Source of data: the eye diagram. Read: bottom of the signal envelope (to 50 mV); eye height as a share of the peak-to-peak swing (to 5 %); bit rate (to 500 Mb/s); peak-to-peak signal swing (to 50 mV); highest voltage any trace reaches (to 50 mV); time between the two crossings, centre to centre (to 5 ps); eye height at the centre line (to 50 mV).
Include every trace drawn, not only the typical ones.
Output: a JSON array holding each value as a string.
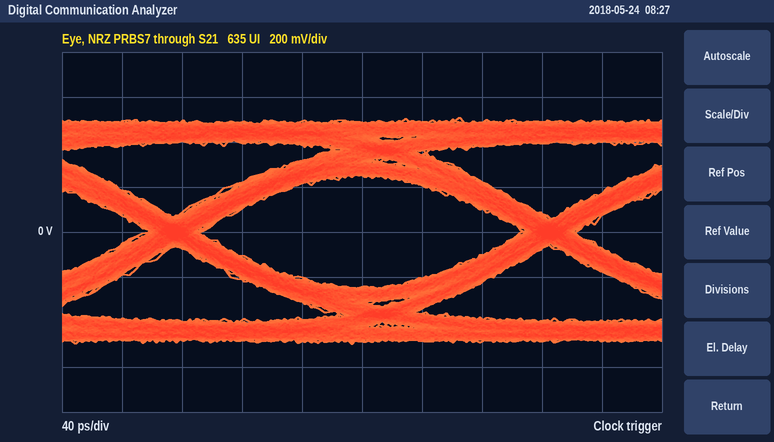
["-500 mV", "50 %", "4.0 Gb/s", "1.00 V", "500 mV", "250 ps", "500 mV"]
